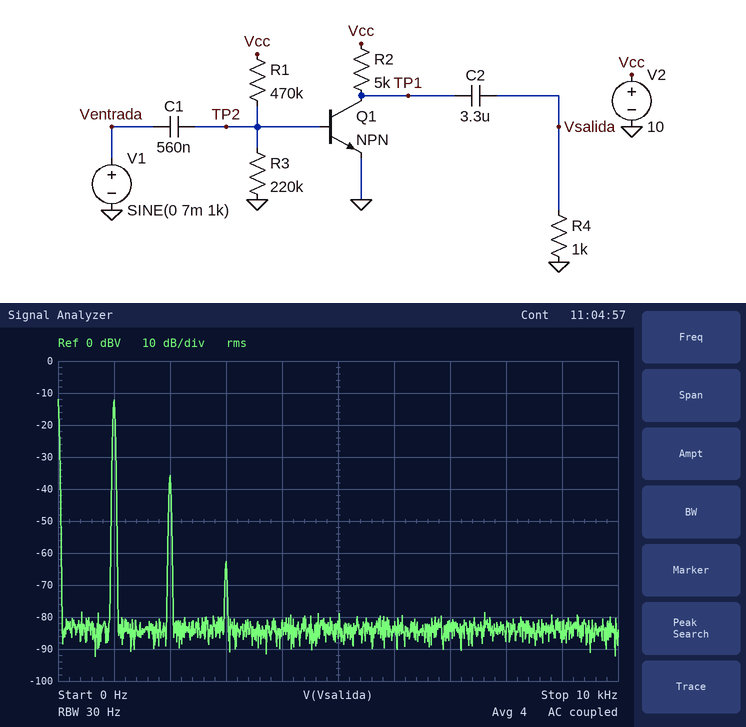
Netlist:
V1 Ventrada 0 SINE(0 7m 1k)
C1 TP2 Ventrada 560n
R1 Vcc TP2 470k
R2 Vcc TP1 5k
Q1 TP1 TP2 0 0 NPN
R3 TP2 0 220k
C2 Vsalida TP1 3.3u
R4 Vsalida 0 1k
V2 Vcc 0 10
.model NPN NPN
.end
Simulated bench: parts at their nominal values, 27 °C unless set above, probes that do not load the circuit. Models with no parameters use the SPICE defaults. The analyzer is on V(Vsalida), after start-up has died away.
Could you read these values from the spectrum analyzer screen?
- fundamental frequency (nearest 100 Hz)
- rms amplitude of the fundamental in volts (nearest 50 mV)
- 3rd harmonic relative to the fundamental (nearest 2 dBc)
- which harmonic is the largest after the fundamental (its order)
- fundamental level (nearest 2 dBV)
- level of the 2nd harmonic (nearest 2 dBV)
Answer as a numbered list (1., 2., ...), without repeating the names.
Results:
1. 1.0 kHz
2. 250 mV
3. -50 dBc
4. 2
5. -12 dBV
6. -36 dBV
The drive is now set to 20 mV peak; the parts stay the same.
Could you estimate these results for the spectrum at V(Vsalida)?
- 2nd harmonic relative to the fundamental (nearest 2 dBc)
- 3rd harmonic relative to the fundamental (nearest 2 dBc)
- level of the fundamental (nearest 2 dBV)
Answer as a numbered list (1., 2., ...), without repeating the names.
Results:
1. -14 dBc
2. -32 dBc
3. -4 dBV
